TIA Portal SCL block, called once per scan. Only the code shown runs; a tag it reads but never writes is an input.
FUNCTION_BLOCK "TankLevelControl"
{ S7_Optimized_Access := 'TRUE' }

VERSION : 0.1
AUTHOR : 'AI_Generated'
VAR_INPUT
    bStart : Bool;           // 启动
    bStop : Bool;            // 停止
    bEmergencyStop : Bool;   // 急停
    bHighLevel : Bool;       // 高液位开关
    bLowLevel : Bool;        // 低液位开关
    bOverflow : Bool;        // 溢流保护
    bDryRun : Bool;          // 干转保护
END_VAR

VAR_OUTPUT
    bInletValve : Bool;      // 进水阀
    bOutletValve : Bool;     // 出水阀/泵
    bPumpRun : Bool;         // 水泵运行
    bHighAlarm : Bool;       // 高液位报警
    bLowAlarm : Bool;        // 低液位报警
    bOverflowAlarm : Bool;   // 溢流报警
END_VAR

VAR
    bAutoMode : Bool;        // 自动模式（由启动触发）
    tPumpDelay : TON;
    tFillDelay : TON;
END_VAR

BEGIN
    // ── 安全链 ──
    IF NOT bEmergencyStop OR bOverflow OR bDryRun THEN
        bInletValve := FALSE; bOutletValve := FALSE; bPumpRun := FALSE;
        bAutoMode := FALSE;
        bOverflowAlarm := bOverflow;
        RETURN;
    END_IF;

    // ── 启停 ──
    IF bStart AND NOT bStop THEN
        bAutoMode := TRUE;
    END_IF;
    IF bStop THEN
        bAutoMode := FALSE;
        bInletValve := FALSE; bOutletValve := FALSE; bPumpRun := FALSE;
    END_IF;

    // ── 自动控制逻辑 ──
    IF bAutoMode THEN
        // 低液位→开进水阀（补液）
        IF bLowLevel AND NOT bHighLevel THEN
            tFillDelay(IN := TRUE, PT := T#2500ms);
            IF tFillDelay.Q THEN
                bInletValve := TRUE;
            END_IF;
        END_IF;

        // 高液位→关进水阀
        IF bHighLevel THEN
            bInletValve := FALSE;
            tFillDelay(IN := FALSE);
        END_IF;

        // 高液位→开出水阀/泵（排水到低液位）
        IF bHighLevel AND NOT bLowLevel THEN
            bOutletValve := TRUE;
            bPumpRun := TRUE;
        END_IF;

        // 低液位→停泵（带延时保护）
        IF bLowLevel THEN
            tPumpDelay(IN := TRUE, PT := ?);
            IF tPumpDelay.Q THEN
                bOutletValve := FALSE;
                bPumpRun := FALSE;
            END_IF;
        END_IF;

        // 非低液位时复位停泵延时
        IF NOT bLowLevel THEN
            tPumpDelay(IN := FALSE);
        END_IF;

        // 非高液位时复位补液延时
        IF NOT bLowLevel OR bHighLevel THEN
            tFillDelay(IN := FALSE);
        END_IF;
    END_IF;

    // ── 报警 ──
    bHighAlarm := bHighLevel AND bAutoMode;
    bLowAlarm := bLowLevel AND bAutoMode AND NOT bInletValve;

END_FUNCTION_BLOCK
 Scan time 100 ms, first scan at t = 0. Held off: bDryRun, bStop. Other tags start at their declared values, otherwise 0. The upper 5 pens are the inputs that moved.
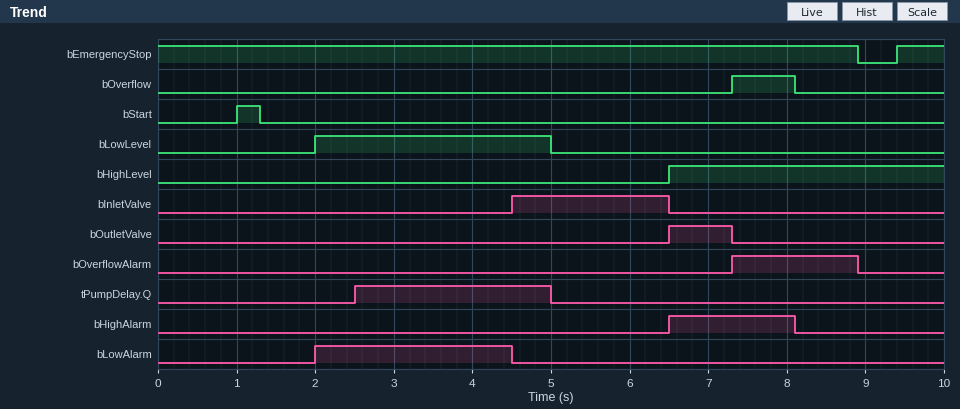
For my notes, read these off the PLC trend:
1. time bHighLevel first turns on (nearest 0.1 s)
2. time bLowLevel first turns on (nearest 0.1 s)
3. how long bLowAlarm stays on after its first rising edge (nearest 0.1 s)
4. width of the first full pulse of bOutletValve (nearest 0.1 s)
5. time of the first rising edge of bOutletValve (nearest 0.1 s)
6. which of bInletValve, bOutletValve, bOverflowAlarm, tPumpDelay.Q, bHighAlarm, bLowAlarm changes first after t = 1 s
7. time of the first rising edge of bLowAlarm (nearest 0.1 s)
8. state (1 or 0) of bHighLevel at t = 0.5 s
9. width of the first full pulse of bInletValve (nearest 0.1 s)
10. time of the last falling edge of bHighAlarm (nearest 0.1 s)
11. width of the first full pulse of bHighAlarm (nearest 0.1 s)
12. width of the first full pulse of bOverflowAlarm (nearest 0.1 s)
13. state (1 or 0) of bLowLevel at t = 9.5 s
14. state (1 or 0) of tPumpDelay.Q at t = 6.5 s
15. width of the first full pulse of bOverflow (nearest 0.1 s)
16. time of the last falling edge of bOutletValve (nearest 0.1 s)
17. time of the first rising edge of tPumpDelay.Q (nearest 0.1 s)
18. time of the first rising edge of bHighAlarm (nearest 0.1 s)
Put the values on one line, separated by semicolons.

6.5 s; 2.0 s; 2.5 s; 0.8 s; 6.5 s; bLowAlarm; 2.0 s; 0; 2.0 s; 8.1 s; 1.6 s; 1.6 s; 0; 0; 0.8 s; 7.3 s; 2.5 s; 6.5 s
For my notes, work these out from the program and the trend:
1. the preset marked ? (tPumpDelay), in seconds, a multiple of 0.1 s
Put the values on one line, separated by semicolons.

0.5 s
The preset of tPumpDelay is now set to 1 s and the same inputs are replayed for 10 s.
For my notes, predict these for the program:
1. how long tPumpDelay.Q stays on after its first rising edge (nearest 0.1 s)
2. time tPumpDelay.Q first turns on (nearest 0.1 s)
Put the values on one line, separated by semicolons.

2.0 s; 3.0 s
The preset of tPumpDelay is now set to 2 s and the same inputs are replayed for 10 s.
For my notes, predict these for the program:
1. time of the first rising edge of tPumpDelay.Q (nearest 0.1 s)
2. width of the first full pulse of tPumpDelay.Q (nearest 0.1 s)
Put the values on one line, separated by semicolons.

4.0 s; 1.0 s
